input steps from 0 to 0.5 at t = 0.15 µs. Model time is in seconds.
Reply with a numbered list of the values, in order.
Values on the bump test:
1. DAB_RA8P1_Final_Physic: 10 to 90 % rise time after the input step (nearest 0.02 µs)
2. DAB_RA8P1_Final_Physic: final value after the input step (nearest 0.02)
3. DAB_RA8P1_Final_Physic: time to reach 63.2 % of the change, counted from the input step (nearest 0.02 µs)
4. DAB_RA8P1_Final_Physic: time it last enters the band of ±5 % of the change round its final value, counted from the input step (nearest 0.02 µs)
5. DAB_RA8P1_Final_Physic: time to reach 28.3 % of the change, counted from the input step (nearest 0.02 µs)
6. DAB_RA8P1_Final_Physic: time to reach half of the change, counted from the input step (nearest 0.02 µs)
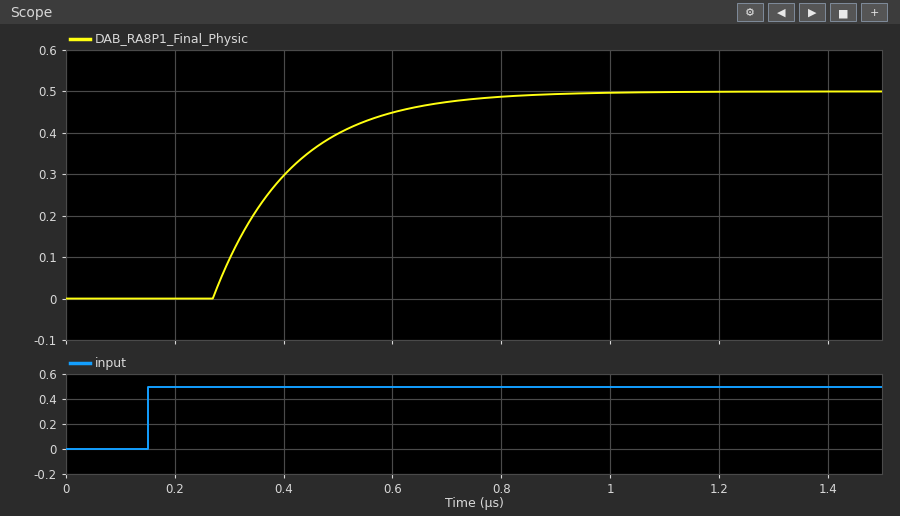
1. 0.32 µs
2. 0.50
3. 0.26 µs
4. 0.56 µs
5. 0.16 µs
6. 0.22 µs
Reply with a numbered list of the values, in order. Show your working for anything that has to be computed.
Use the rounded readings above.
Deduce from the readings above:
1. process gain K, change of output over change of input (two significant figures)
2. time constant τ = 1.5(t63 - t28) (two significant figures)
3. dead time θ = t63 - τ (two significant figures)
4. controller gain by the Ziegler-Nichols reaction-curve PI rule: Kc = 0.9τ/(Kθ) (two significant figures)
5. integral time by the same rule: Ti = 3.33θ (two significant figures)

1. (0.5 - 0) / 0.5 = 1.0
2. 1.5 × (0.26 - 0.16) = 0.15 µs
3. 0.26 - 0.15 = 0.11 µs
4. 0.9 × 0.15 / (1 × 0.11) = 1.2
5. 3.33 × 0.11 = 0.37 µs
